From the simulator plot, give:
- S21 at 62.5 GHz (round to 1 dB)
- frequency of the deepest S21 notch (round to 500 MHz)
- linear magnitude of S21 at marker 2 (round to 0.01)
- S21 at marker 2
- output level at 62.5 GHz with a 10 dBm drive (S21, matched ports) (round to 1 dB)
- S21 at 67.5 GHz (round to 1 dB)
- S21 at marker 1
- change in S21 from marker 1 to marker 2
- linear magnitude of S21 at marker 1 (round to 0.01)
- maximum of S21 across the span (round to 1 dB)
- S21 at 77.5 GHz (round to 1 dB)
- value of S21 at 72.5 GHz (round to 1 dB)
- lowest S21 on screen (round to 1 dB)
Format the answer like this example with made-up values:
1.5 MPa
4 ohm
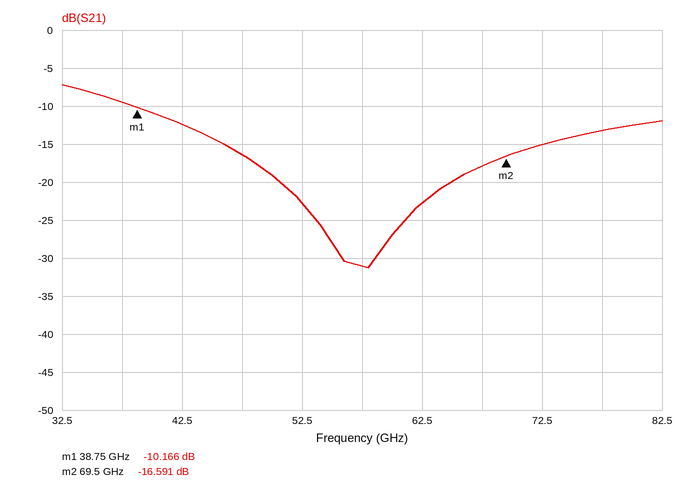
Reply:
-23 dB
58.0 GHz
0.15
-16.591 dB
-13 dBm
-18 dB
-10.166 dB
-6.425 dB
0.31
-7 dB
-13 dB
-15 dB
-31 dB
